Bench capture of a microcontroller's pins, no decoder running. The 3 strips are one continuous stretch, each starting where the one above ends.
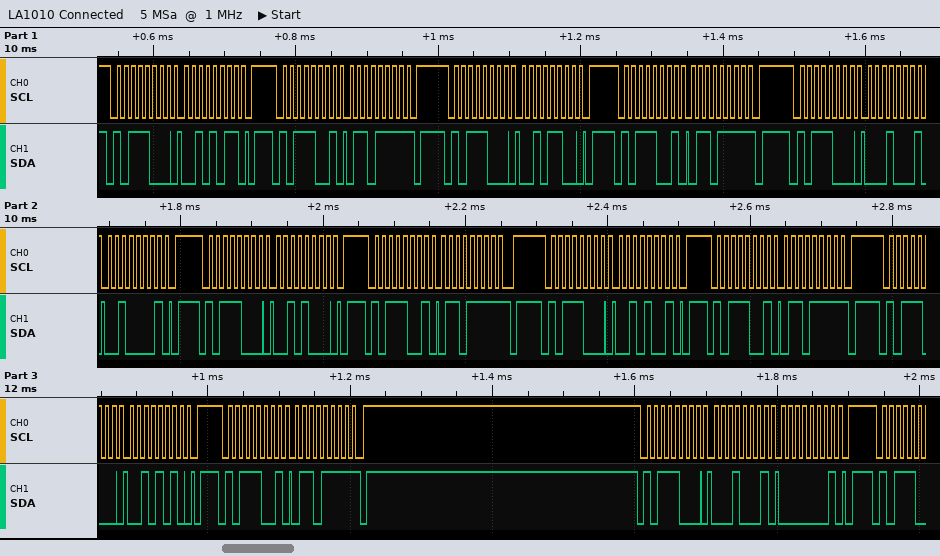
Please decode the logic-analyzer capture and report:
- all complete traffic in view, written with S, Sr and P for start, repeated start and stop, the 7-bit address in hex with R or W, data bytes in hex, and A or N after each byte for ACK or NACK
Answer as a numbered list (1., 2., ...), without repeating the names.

1. S 5CW A 2B A P S 5CR A 6F N P S 5CW A 2C A P S 5CR A 6F N P S 5CW A 11 A 21 A P S 5CW A 28 A P S 5CR A 6F N P S 5CW A 29 A P S 5CR A 6F N P S 5CW A 2A A P S 5CR A 6F N P S 5CW A 11 A 01 A P
